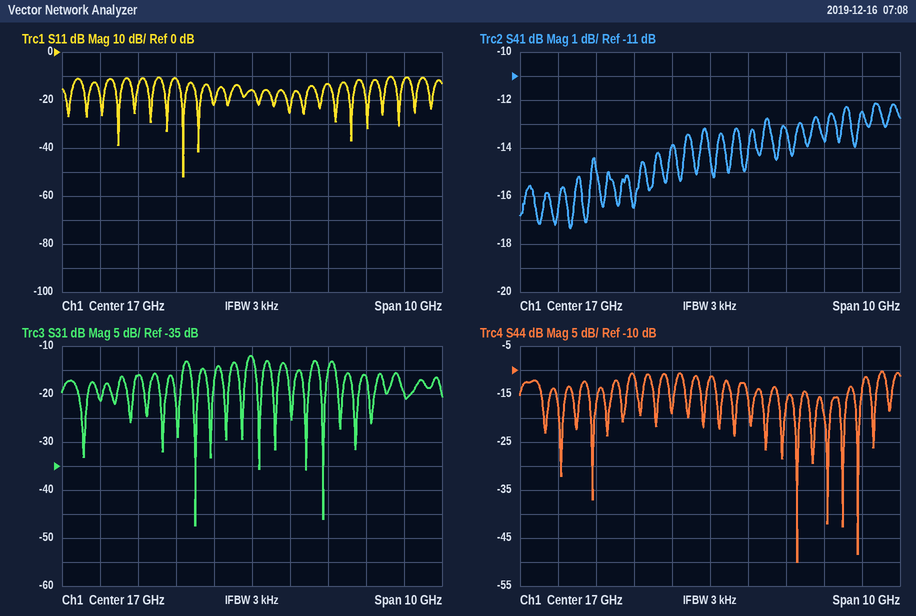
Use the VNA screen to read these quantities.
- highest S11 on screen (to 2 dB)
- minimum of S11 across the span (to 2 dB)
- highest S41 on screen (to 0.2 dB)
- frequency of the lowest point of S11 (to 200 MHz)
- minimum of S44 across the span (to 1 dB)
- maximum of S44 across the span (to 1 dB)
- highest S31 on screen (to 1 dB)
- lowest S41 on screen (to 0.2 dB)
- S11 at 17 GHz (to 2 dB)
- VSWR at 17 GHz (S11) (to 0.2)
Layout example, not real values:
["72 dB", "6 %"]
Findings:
["-10 dB", "-52 dB", "-12.2 dB", "15.2 GHz", "-50 dB", "-10 dB", "-12 dB", "-17.4 dB", "-16 dB", "1.4"]
